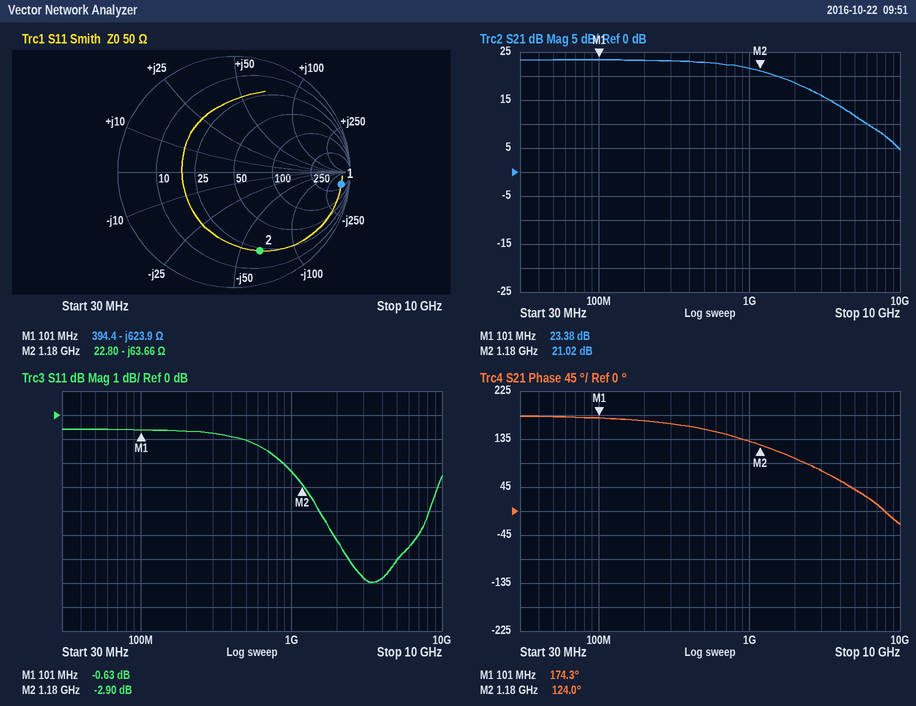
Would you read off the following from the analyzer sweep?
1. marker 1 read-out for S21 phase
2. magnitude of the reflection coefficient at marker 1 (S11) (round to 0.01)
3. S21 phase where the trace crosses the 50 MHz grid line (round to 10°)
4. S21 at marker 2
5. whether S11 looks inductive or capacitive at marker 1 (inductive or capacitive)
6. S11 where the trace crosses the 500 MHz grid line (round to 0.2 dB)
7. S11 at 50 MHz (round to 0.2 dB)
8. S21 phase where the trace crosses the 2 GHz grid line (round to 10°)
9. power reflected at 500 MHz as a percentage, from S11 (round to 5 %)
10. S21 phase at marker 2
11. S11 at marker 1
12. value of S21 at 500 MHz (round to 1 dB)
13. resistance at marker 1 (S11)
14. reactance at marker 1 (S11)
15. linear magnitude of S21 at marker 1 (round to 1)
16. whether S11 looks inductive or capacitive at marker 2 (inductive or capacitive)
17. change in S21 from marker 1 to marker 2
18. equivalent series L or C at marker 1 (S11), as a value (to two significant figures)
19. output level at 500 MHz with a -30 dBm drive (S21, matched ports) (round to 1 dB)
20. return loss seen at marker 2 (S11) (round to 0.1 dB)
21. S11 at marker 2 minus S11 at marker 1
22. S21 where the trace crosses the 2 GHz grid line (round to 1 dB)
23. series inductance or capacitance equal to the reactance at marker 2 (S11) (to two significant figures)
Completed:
174.3°
0.93
180°
21.02 dB
capacitive
-1.0 dB
-0.6 dB
100°
80 %
124.0°
-0.63 dB
23 dB
394.4 Ω
-623.9 Ω
15
capacitive
-2.36 dB
2.5 pF
-7 dBm
2.9 dB
-2.27 dB
19 dB
2.1 pF
